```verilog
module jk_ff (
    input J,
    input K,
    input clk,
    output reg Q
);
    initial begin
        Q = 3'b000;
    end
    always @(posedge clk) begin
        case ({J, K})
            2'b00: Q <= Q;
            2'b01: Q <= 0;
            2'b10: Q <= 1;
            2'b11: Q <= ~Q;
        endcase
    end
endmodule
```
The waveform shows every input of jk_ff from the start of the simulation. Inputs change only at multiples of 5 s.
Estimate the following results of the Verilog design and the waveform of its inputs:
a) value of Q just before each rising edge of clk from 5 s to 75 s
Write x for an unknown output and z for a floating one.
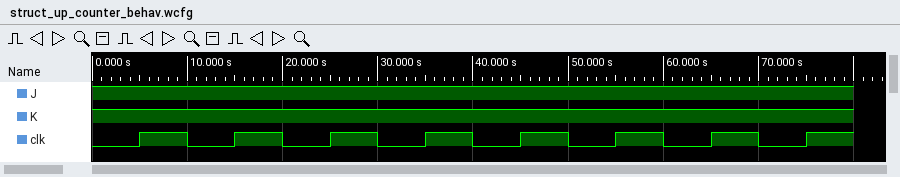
0 1 0 1 0 1 0 1
